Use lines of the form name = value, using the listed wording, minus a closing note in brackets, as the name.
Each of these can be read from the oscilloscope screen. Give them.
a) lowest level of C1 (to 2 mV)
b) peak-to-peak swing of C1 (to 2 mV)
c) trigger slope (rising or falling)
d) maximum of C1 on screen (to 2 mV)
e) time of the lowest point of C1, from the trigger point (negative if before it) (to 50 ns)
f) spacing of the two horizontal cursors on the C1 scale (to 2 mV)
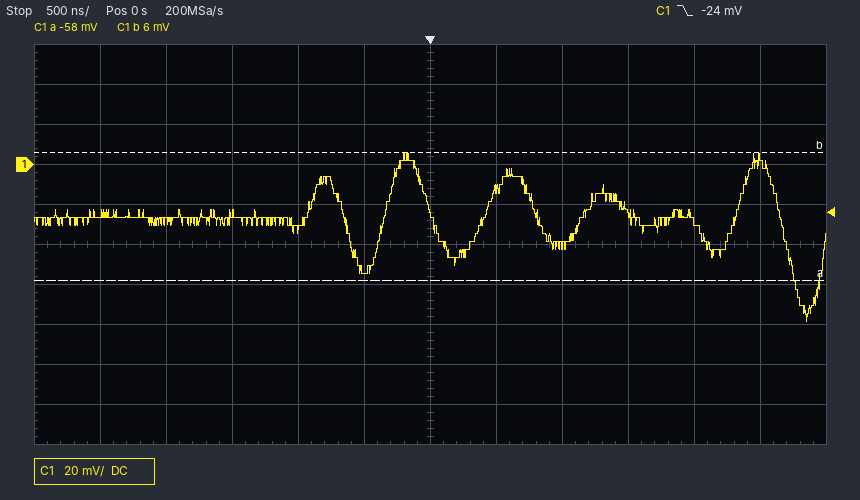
lowest level of C1 = -78 mV
peak-to-peak swing of C1 = 84 mV
trigger slope = falling
maximum of C1 on screen = 6 mV
time of the lowest point of C1, from the trigger point (negative if before it) = +2.85 µs
spacing of the two horizontal cursors on the C1 scale = 64 mV
